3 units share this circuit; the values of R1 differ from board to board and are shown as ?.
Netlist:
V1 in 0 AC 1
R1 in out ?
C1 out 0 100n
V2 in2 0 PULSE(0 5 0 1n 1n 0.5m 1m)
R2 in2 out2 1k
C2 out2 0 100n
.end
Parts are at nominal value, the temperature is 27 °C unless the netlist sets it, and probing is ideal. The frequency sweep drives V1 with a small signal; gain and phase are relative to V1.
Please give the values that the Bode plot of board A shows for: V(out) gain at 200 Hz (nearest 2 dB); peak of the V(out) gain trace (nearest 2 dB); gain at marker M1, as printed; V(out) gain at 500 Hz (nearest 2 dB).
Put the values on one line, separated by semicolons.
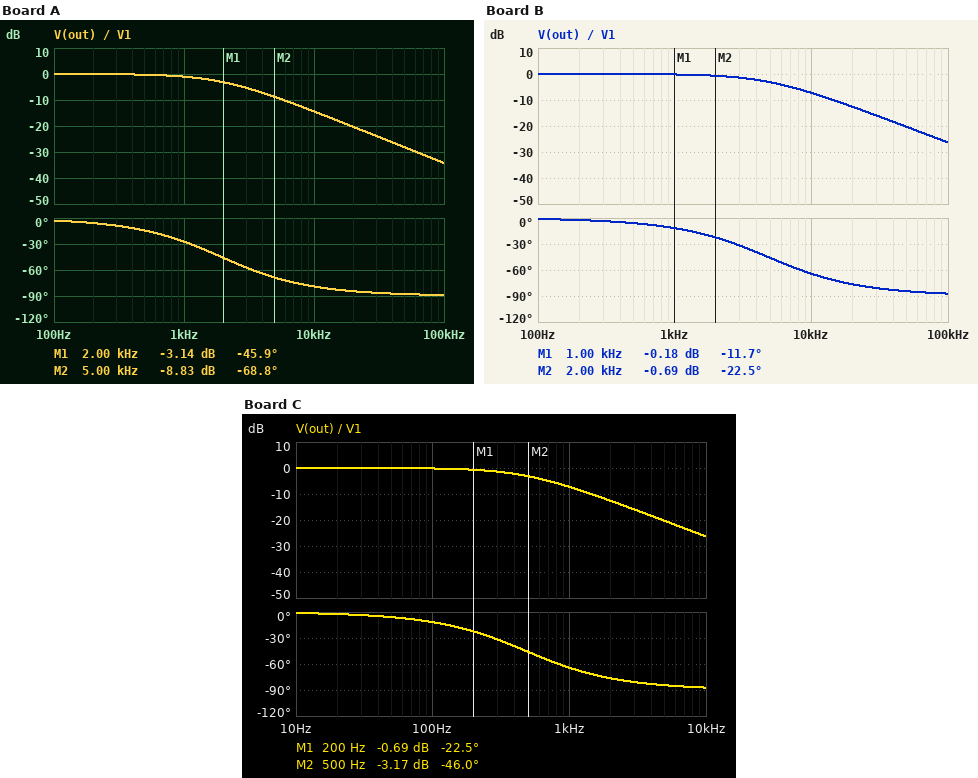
0 dB; 0 dB; -3.14 dB; 0 dB
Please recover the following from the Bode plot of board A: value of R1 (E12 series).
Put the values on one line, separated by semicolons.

820 Ω
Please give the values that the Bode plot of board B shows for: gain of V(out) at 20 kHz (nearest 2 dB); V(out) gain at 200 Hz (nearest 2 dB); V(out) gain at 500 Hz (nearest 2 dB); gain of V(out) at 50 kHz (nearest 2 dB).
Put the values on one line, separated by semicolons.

-12 dB; 0 dB; 0 dB; -20 dB
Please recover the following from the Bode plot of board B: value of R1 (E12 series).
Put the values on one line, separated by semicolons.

330 Ω
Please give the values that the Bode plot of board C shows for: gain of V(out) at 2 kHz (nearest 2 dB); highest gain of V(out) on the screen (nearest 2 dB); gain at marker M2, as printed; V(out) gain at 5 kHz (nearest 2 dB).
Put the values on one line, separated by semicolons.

-12 dB; 0 dB; -3.17 dB; -20 dB
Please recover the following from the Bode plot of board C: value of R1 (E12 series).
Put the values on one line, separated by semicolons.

3.3 kΩ
